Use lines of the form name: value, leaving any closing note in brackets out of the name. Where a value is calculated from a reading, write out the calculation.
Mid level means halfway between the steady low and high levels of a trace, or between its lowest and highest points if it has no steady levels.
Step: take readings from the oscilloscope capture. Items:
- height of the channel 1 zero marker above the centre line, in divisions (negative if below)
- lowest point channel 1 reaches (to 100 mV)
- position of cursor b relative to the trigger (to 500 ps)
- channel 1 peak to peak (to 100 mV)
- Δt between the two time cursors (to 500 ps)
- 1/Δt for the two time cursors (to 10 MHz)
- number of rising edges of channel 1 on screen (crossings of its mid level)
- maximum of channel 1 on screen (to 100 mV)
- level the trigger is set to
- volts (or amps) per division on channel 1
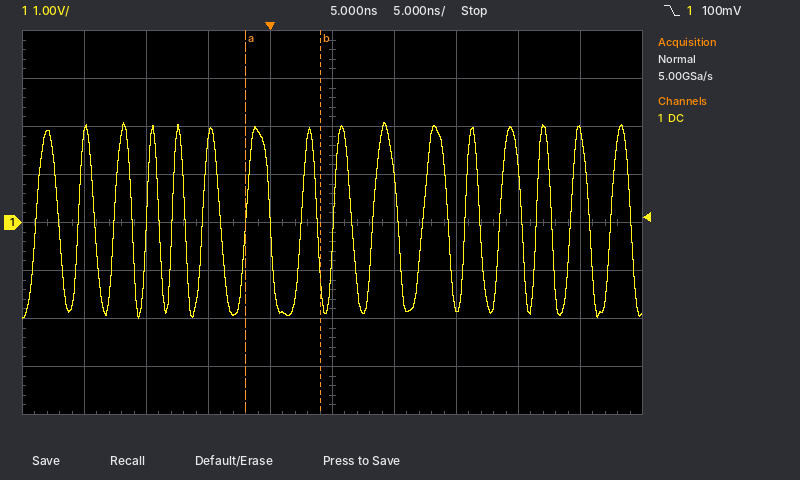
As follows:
height of the channel 1 zero marker above the centre line, in divisions: 0.0 div
lowest point channel 1 reaches: -2.0 V
position of cursor b relative to the trigger: +4.0 ns
channel 1 peak to peak: 2.1 V − (-2.0 V) = 4.1 V
Δt between the two time cursors: 6.0 ns
1/Δt for the two time cursors: 1 / 6.0 ns ≈ 170 MHz
number of rising edges of channel 1 on screen: 16
maximum of channel 1 on screen: 2.1 V
level the trigger is set to: 100 mV
volts (or amps) per division on channel 1: 1 V
